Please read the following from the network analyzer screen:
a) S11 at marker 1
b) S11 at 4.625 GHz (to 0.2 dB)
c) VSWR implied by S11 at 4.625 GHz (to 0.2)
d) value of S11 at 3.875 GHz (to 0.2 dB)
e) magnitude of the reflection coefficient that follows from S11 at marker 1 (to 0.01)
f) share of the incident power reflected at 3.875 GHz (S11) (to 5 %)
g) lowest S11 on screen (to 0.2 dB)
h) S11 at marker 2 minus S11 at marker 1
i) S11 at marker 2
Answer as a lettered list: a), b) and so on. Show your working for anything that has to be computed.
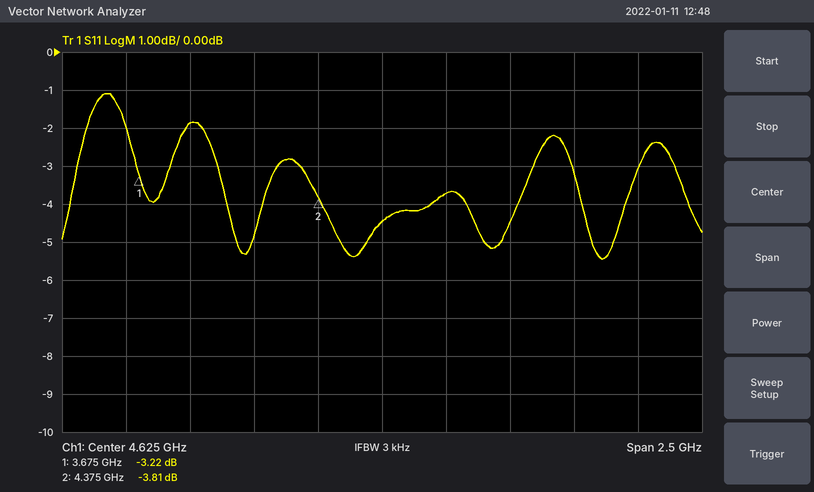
a) -3.22 dB
b) -4.4 dB
c) |Γ| = 10^(-4.4/20) = 0.6026; VSWR = (1 + 0.6026)/(1 − 0.6026) ≈ 4.0
d) -1.8 dB
e) 10^(-3.22/20) ≈ 0.69
f) 10^(-1.8/10) ≈ 66.1 %, so 65 % to the nearest 5 %
g) -5.4 dB
h) -3.81 − (-3.22) = -0.59 dB
i) -3.81 dB
